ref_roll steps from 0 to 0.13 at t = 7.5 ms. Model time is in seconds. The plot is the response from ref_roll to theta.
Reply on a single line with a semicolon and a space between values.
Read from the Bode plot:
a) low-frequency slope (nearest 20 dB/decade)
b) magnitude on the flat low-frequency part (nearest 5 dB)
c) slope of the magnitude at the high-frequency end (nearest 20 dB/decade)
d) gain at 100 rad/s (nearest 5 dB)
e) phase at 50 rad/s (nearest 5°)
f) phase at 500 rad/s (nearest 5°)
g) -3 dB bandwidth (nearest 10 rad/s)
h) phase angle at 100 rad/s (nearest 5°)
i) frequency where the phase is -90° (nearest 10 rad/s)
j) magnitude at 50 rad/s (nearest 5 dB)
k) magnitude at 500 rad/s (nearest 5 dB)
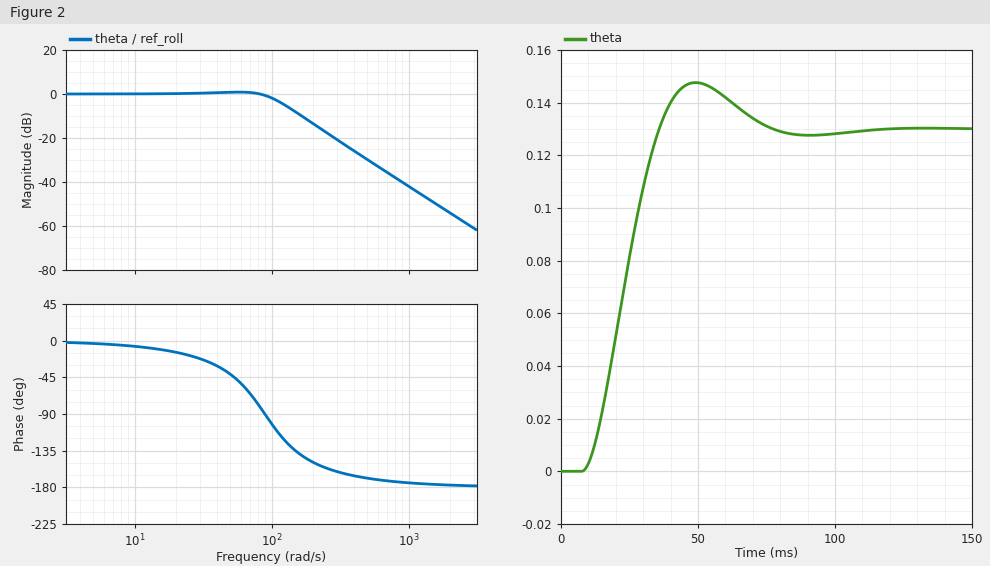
0 dB/decade; 0 dB; -40 dB/decade; 0 dB; -40°; -170°; 110 rad/s; -100°; 90 rad/s; 0 dB; -30 dB
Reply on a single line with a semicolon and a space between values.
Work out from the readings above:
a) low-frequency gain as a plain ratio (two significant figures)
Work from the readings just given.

1.0
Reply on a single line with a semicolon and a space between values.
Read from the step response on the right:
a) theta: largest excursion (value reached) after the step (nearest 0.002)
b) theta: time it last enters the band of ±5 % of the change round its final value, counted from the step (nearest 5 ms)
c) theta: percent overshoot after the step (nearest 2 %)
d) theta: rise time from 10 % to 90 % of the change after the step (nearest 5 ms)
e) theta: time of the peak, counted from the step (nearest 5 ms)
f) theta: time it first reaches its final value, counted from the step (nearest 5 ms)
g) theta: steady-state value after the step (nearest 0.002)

0.148; 60 ms; 14 %; 20 ms; 40 ms; 30 ms; 0.130
